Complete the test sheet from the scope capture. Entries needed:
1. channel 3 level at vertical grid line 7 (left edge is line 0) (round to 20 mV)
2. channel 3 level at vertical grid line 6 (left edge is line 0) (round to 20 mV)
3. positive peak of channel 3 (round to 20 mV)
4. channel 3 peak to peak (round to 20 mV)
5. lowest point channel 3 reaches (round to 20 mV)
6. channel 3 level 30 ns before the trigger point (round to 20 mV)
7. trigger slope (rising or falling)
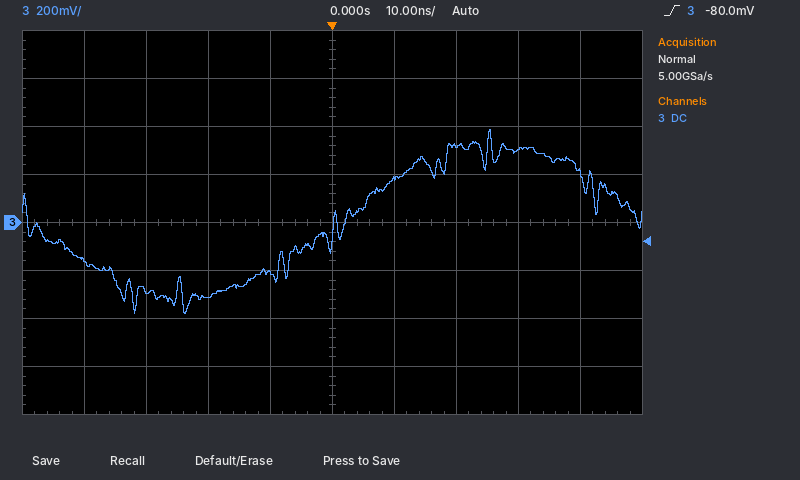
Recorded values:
320 mV
180 mV
380 mV
760 mV
-380 mV
-280 mV
rising
